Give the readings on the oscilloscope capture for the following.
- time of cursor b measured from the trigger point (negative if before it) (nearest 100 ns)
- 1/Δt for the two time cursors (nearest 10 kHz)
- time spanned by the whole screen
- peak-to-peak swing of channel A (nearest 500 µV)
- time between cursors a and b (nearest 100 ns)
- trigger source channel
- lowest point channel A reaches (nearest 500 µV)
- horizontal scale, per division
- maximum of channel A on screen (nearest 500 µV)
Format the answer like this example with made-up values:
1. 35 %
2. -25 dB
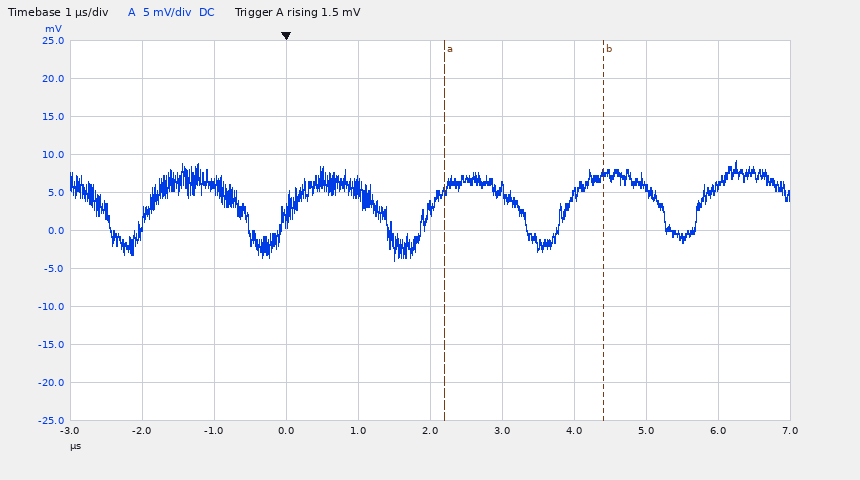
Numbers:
1. +4.4 µs
2. 450 kHz
3. 10 µs
4. 13.0 mV
5. 2.2 µs
6. channel A
7. -4.0 mV
8. 1 µs
9. 9.0 mV
